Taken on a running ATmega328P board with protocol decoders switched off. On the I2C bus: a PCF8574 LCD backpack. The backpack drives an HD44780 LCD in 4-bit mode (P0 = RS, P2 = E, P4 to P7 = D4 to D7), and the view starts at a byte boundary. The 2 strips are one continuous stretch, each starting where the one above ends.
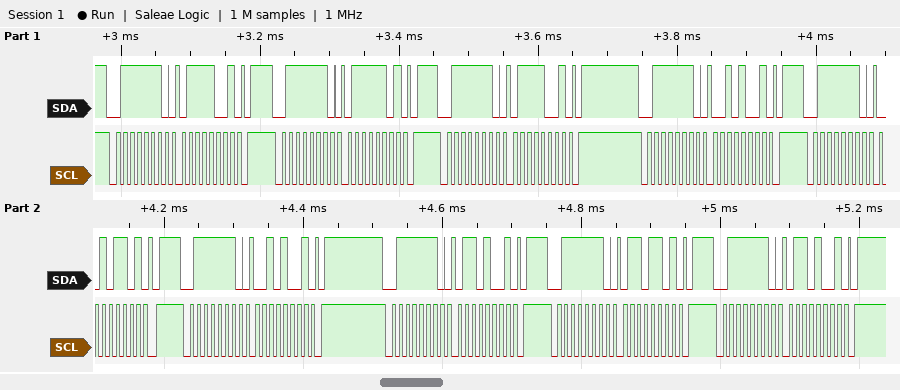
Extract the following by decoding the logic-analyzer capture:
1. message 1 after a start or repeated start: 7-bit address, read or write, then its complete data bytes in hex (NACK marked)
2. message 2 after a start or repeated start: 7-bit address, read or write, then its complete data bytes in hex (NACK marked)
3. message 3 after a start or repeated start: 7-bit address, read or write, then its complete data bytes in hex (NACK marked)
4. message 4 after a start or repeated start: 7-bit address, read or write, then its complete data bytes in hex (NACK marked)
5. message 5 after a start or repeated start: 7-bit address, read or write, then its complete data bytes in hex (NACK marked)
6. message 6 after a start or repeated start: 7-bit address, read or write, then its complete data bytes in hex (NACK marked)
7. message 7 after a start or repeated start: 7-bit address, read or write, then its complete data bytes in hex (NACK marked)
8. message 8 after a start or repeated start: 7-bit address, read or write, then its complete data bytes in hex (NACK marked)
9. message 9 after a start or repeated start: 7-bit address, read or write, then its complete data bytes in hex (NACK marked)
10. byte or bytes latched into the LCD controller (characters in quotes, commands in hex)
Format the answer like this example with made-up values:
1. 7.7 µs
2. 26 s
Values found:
1. 0x3F write: 79
2. 0x3F write: 7D
3. 0x3F write: 79
4. 0x3F write: 29
5. 0x3F write: 2D
6. 0x3F write: 29
7. 0x3F write: 69
8. 0x3F write: 6D
9. 0x3F write: 69
10. 'r'
